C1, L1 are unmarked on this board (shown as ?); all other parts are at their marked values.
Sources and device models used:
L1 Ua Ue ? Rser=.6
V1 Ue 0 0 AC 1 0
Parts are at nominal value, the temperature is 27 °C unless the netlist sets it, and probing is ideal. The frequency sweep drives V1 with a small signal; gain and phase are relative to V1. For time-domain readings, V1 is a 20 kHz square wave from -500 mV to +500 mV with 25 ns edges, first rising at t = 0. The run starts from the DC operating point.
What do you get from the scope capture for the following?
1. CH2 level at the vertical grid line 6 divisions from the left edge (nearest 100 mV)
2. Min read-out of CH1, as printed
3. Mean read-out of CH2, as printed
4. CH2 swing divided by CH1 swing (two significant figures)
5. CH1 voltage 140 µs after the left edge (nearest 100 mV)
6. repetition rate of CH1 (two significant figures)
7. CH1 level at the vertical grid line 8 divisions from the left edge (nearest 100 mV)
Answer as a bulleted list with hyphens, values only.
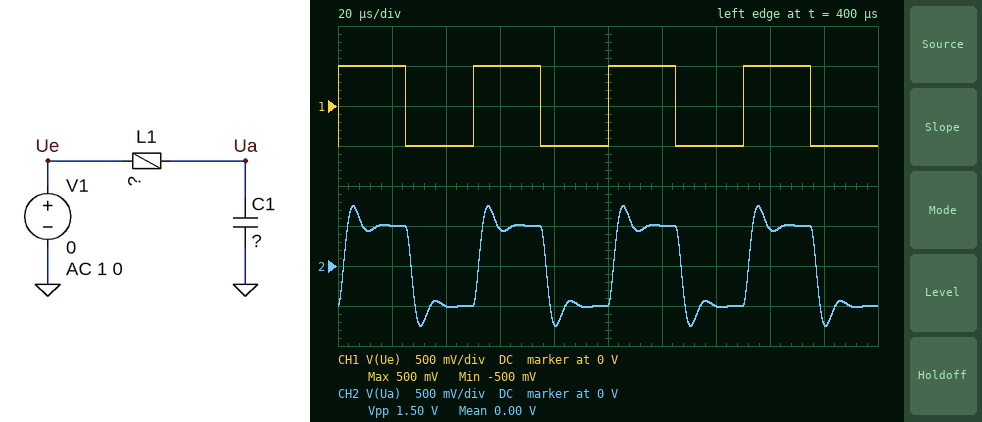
- 500 mV
- -500 mV
- 0.00 V
- 1.5
- -500 mV
- 20 kHz
- 500 mV
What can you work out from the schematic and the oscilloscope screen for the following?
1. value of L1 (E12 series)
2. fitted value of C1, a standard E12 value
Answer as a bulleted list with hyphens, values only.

- 1.2 µH
- 2.2 µF
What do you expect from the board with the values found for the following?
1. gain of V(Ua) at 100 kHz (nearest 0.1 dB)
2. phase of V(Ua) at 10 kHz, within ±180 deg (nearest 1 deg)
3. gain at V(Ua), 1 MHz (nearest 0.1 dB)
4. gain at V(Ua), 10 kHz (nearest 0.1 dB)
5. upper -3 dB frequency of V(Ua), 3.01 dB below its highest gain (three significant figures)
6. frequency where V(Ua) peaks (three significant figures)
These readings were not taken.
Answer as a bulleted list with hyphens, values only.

- 1.6 dB
- -5 deg
- -40.3 dB
- 0.1 dB
- 116 kHz
- 80.2 kHz
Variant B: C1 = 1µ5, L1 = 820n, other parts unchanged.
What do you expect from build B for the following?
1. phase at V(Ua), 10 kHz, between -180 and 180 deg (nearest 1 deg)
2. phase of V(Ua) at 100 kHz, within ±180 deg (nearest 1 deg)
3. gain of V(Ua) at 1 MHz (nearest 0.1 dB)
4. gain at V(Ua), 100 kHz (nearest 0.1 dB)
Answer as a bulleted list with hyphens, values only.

- -3 deg
- -48 deg
- -33.6 dB
- 2.3 dB
